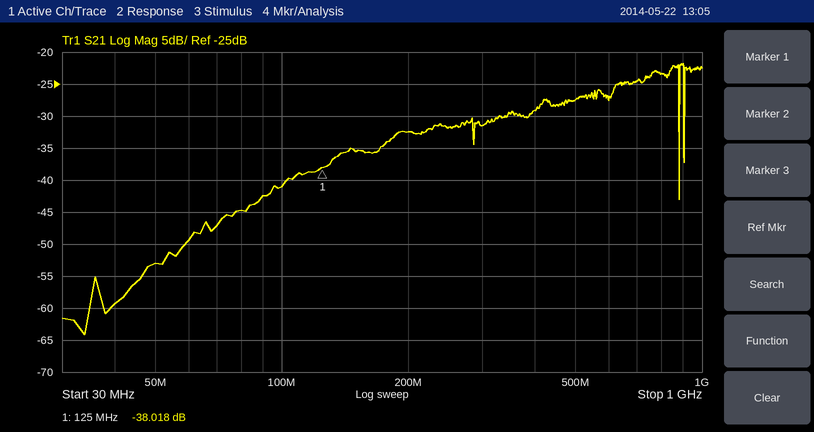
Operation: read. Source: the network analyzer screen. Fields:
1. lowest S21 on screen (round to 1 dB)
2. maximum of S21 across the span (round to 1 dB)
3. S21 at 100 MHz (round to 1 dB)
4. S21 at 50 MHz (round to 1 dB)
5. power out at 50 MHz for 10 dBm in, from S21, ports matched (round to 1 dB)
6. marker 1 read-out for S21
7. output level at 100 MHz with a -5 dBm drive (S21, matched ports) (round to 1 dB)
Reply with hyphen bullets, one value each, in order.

- -64 dB
- -22 dB
- -41 dB
- -53 dB
- -43 dBm
- -38.018 dB
- -46 dBm
